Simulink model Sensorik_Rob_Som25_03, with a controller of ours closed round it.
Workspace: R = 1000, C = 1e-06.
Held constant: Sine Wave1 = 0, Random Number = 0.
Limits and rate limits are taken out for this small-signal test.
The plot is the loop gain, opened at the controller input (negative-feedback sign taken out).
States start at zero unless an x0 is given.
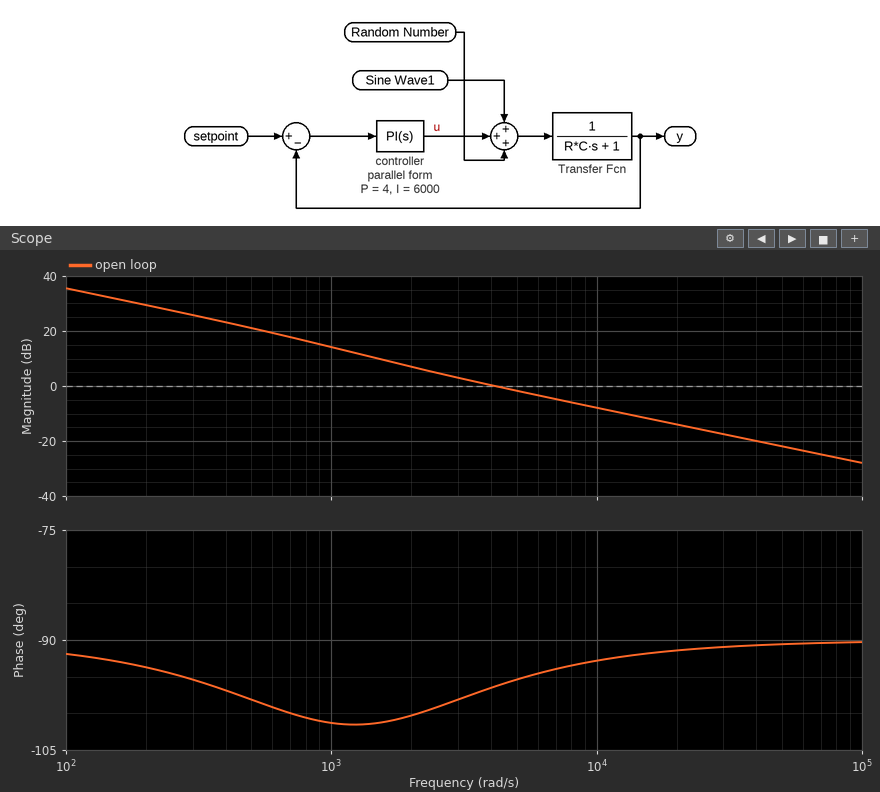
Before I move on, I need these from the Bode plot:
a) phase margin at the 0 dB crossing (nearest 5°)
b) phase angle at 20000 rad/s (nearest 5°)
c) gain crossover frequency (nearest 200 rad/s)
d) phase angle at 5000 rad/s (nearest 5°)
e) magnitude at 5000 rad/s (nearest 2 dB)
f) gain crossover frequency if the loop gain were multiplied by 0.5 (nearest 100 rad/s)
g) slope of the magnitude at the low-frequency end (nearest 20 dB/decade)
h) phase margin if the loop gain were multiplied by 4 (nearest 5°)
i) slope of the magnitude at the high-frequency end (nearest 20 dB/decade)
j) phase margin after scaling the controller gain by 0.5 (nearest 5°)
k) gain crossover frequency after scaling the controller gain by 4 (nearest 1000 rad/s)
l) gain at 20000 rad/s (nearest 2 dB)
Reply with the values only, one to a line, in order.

85°
-90°
4200 rad/s
-95°
-2 dB
2200 rad/s
-20 dB/decade
90°
-20 dB/decade
80°
16000 rad/s
-14 dB
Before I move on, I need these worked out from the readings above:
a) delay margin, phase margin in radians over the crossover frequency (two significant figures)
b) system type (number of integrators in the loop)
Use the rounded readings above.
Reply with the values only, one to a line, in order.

0.00035 s
1
